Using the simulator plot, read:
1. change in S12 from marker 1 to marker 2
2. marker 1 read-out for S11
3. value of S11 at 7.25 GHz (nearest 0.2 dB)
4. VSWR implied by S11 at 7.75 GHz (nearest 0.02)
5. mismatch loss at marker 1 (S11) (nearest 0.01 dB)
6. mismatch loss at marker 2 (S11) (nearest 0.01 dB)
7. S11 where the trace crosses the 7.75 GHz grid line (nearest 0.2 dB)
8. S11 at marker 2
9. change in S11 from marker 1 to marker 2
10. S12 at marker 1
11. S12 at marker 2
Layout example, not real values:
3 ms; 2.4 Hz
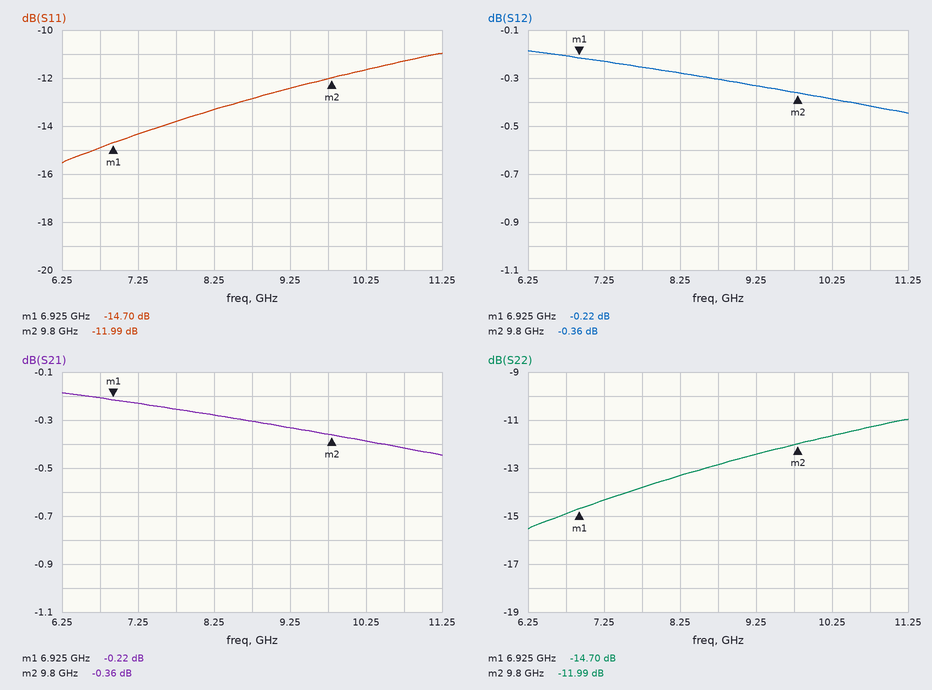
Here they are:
-0.14 dB; -14.70 dB; -14.4 dB; 1.52; 0.15 dB; 0.28 dB; -13.8 dB; -11.99 dB; 2.71 dB; -0.22 dB; -0.36 dB
